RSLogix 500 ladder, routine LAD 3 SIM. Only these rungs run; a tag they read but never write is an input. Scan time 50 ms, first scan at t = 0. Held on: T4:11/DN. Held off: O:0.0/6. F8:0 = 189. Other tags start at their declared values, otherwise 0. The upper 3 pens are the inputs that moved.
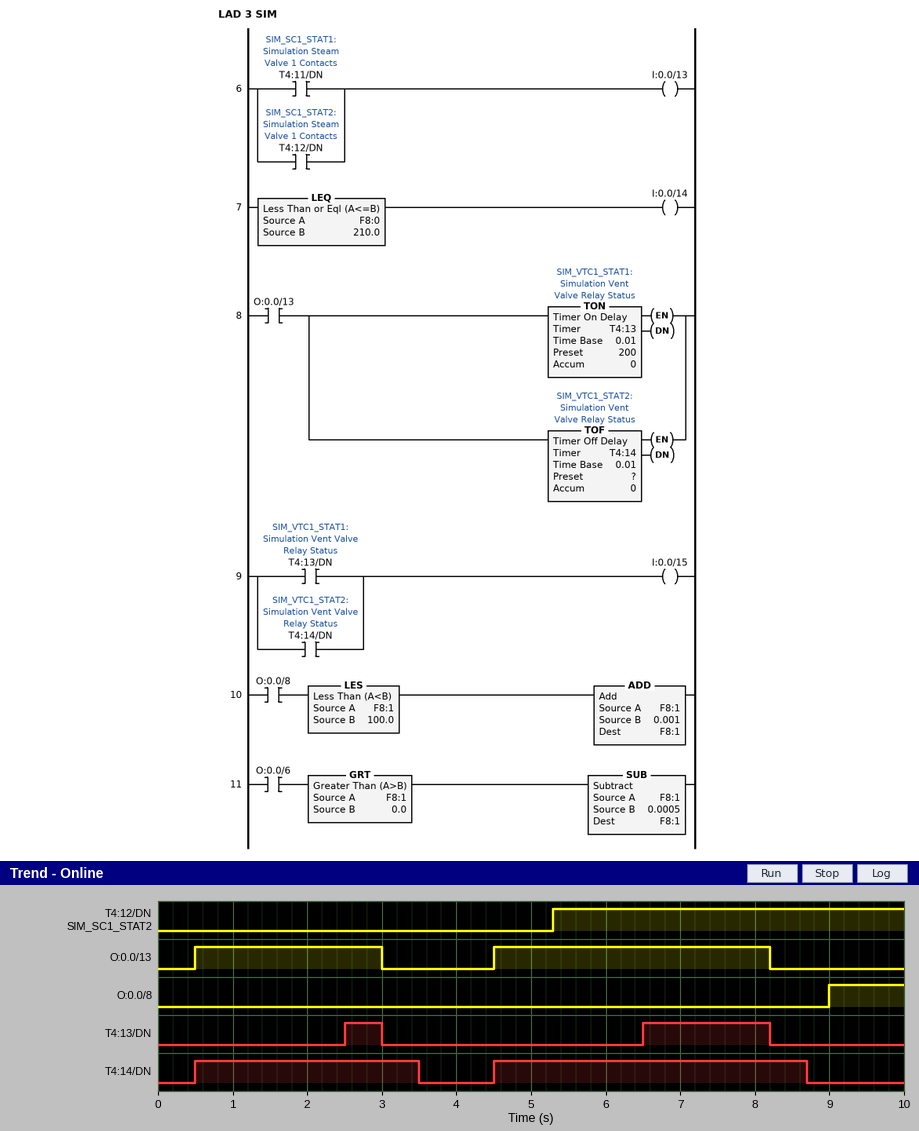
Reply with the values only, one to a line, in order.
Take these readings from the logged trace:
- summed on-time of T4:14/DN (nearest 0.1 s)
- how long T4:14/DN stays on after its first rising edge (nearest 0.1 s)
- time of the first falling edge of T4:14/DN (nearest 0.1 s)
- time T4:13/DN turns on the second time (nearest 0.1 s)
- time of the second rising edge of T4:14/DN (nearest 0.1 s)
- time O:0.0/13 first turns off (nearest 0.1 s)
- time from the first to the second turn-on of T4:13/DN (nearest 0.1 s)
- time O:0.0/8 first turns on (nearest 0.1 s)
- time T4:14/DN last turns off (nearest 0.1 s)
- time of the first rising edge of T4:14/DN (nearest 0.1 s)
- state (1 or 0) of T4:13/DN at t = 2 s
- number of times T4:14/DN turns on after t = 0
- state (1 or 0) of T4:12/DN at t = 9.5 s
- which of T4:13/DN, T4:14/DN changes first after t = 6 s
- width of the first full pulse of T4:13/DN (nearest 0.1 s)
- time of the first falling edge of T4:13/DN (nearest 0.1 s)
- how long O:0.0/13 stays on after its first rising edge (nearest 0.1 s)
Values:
7.2 s
3.0 s
3.5 s
6.5 s
4.5 s
3.0 s
4.0 s
9.0 s
8.7 s
0.5 s
0
2
1
T4:13/DN
0.5 s
3.0 s
2.5 s
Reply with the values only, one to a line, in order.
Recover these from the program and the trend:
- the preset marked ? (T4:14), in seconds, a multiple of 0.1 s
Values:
0.5 s
